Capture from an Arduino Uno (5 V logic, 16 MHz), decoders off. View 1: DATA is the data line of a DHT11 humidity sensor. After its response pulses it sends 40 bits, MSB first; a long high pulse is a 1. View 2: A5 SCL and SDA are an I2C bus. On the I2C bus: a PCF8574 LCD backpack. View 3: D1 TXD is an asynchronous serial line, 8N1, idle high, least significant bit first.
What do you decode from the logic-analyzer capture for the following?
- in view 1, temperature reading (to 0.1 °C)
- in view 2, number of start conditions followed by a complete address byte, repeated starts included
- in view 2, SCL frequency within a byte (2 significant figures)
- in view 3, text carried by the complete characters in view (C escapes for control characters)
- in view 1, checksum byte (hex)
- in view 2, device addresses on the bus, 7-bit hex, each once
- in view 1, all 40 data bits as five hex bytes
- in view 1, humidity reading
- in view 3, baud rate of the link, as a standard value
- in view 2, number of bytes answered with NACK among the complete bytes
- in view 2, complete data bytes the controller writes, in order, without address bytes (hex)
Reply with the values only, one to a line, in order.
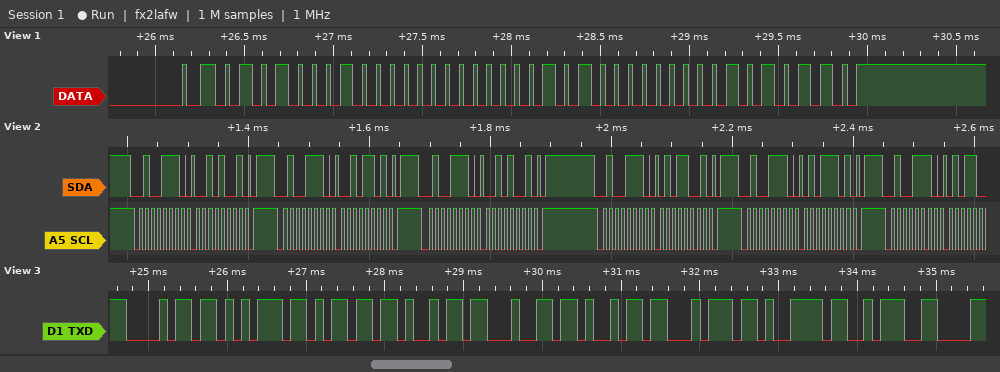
5.0 °C
6
100 kHz
"humidity:"
0x56
0x27
51 00 05 00 56
81 %
9600 baud
0
29 2D 29 59 5D
